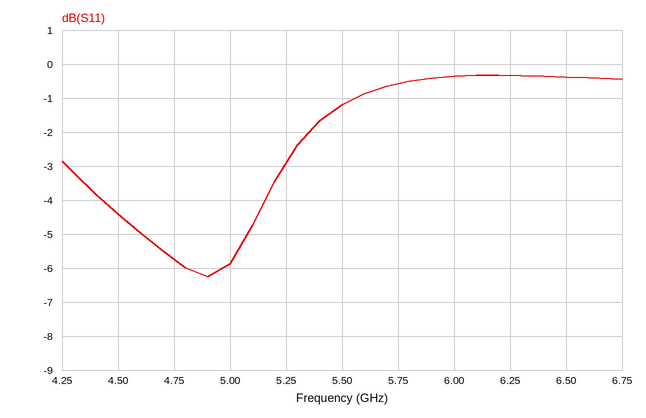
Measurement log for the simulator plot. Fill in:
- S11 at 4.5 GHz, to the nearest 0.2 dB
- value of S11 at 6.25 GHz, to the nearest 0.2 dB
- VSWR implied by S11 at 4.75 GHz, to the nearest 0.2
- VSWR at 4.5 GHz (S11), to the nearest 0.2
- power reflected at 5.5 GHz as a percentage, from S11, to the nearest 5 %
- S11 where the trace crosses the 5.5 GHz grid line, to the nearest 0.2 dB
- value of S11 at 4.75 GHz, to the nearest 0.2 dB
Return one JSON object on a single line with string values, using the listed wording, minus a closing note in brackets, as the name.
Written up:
{"S11 at 4.5 GHz, to the nearest 0.2 dB": "-4.4 dB", "value of S11 at 6.25 GHz, to the nearest 0.2 dB": "-0.4 dB", "VSWR implied by S11 at 4.75 GHz, to the nearest 0.2": "3.2", "VSWR at 4.5 GHz (S11), to the nearest 0.2": "4.0", "power reflected at 5.5 GHz as a percentage, from S11, to the nearest 5 %": "75 %", "S11 where the trace crosses the 5.5 GHz grid line, to the nearest 0.2 dB": "-1.2 dB", "value of S11 at 4.75 GHz, to the nearest 0.2 dB": "-5.8 dB"}
